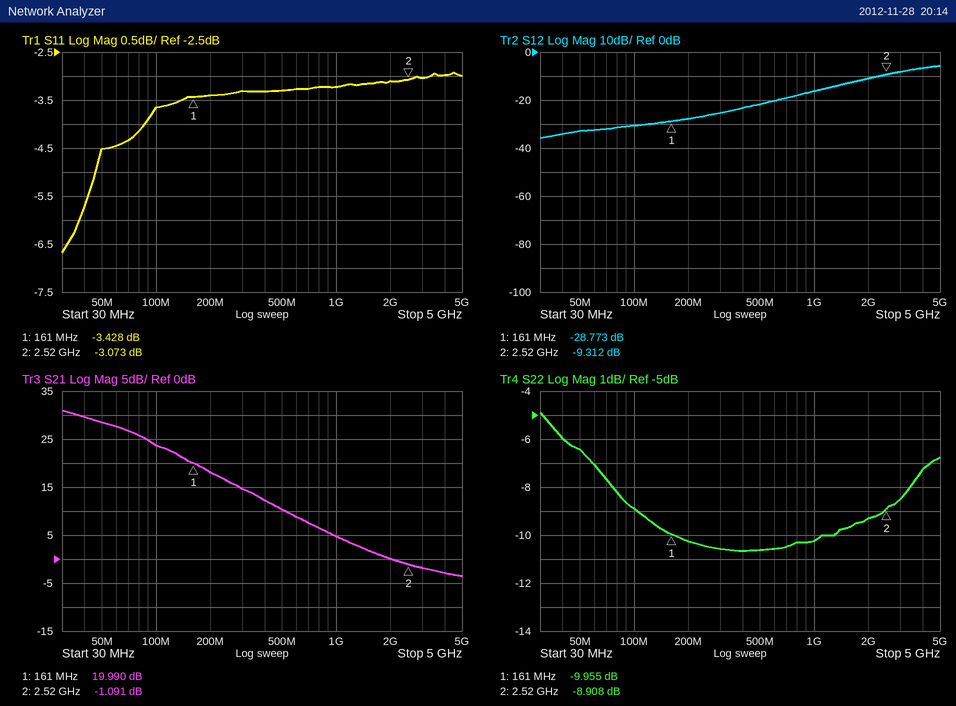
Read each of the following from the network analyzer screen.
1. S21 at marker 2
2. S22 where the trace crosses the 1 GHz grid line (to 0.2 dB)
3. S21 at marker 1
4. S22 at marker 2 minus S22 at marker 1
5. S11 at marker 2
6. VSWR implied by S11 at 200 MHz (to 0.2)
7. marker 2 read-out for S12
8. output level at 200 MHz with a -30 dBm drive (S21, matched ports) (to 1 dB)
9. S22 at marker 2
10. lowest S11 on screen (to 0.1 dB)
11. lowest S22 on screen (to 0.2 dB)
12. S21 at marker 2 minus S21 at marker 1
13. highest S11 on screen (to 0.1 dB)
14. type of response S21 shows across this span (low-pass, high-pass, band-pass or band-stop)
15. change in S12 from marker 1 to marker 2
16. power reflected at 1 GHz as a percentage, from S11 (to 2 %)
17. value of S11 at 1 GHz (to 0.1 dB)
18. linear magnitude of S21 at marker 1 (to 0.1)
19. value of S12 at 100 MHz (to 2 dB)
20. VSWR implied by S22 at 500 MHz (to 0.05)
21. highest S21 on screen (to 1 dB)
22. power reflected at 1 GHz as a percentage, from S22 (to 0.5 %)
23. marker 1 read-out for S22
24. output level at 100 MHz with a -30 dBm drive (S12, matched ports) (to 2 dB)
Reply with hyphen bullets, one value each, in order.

- -1.091 dB
- -10.2 dB
- 19.990 dB
- 1.047 dB
- -3.073 dB
- 5.2
- -9.312 dB
- -12 dBm
- -8.908 dB
- -6.7 dB
- -10.6 dB
- -21.081 dB
- -2.9 dB
- low-pass
- 19.461 dB
- 48 %
- -3.2 dB
- 10.0
- -30 dB
- 1.85
- 31 dB
- 9.5 %
- -9.955 dB
- -60 dBm
